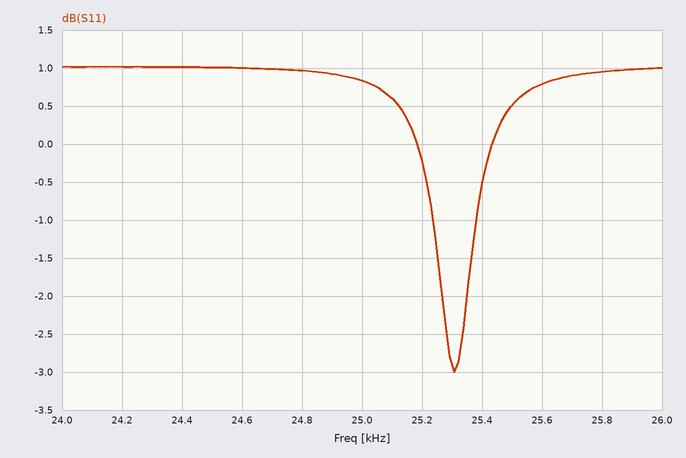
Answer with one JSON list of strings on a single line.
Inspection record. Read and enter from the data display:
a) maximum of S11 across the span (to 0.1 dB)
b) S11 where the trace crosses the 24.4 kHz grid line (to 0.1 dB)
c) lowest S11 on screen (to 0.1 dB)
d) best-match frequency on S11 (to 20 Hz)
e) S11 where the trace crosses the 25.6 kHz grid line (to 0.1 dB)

["1.0 dB", "1.0 dB", "-3.0 dB", "25.30 kHz", "0.8 dB"]
